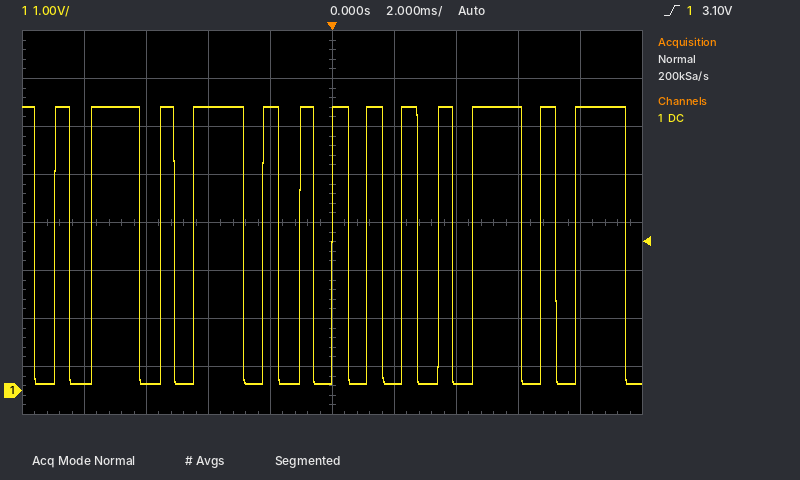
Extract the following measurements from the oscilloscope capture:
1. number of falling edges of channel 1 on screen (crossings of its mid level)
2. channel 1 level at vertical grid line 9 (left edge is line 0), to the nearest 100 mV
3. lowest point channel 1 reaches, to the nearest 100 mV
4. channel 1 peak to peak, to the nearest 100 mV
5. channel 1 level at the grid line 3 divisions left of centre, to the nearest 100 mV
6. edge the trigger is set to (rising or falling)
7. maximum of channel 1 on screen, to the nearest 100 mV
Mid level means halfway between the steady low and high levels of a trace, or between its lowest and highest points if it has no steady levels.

14
5.9 V
100 mV
5.8 V
100 mV
rising
5.9 V
